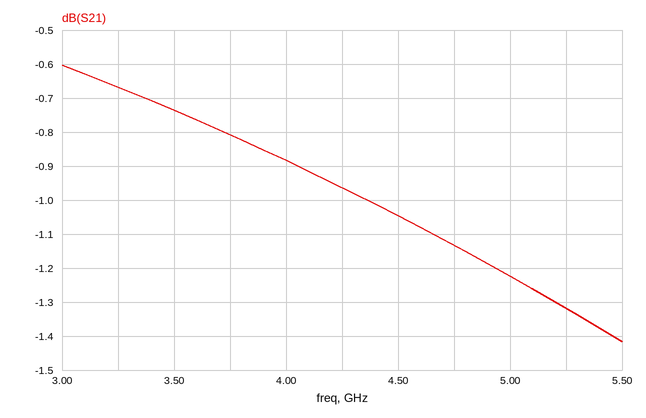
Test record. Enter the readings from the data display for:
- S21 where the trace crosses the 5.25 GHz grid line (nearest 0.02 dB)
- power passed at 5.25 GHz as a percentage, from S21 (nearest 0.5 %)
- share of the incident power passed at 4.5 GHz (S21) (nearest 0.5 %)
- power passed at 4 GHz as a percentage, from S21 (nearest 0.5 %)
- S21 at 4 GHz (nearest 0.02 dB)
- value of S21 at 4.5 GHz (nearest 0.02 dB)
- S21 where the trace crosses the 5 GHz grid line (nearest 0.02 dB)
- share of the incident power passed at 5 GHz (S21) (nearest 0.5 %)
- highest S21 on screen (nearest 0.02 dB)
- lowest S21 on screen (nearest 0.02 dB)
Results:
-1.32 dB
74.0 %
78.5 %
81.5 %
-0.88 dB
-1.04 dB
-1.22 dB
75.5 %
-0.60 dB
-1.42 dB
